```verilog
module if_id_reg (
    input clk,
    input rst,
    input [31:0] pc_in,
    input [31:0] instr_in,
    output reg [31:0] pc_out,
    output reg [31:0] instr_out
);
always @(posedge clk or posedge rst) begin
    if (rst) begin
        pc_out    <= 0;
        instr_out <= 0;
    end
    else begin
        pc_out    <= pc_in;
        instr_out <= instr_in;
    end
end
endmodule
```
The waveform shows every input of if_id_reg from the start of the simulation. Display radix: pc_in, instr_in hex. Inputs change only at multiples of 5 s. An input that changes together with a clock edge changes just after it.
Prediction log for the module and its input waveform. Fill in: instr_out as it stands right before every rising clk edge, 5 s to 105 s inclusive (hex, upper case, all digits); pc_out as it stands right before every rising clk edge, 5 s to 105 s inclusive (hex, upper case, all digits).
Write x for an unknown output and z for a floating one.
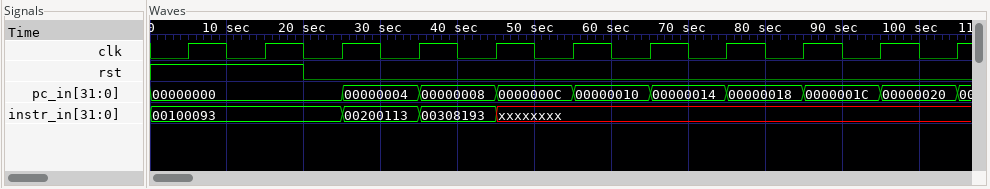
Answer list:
00000000, 00000000, 00000000, 00100093, 00200113, 00308193, x, x, x, x, x
00000000, 00000000, 00000000, 00000000, 00000004, 00000008, 0000000C, 00000010, 00000014, 00000018, 0000001C
